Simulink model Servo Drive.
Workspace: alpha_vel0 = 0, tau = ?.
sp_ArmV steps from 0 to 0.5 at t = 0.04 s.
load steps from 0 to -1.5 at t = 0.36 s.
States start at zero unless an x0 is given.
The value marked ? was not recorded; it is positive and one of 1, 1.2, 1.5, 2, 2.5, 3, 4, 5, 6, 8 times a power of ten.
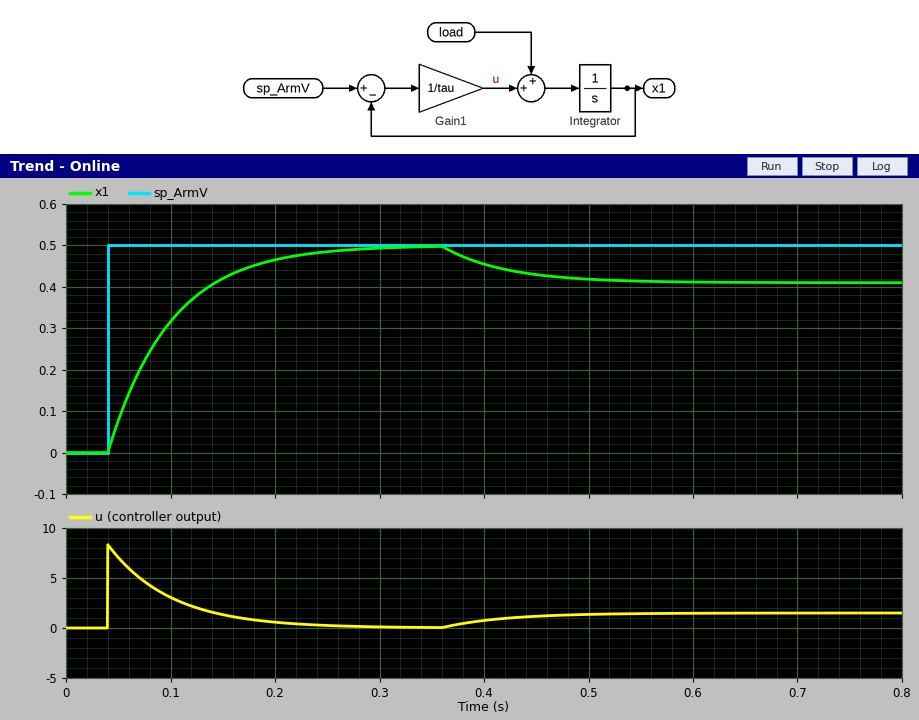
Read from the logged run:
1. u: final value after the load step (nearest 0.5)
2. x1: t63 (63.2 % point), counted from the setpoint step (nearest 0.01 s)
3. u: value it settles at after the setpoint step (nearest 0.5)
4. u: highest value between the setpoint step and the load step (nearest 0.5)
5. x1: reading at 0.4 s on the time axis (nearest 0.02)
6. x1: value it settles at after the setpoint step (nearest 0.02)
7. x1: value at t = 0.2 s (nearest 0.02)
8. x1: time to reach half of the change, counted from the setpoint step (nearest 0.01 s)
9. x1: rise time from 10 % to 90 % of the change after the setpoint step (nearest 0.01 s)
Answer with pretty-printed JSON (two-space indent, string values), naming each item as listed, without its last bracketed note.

{
  "u: final value after the load step": "1.5",
  "x1: t63 (63.2 % point), counted from the setpoint step": "0.06 s",
  "u: value it settles at after the setpoint step": "0.0",
  "u: highest value between the setpoint step and the load step": "8.5",
  "x1: reading at 0.4 s on the time axis": "0.46",
  "x1: value it settles at after the setpoint step": "0.50",
  "x1: value at t = 0.2 s": "0.46",
  "x1: time to reach half of the change, counted from the setpoint step": "0.04 s",
  "x1: rise time from 10 % to 90 % of the change after the setpoint step": "0.13 s"
}
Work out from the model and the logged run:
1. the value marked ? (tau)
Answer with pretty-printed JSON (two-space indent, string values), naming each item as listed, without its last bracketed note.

{
  "the value marked ?": "0.06"
}
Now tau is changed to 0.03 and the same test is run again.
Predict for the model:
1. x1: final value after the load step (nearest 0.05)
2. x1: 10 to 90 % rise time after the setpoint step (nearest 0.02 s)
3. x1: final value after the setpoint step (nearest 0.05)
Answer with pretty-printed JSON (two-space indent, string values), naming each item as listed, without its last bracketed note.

{
  "x1: final value after the load step": "0.45",
  "x1: 10 to 90 % rise time after the setpoint step": "0.06 s",
  "x1: final value after the setpoint step": "0.50"
}
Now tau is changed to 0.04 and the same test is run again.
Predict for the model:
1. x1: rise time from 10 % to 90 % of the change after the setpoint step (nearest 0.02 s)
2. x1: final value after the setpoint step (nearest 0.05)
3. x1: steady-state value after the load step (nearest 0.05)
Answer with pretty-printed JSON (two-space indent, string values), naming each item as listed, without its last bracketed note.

{
  "x1: rise time from 10 % to 90 % of the change after the setpoint step": "0.08 s",
  "x1: final value after the setpoint step": "0.50",
  "x1: steady-state value after the load step": "0.45"
}
